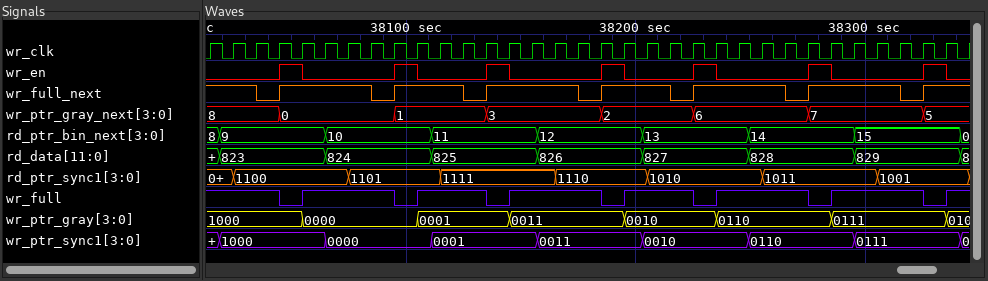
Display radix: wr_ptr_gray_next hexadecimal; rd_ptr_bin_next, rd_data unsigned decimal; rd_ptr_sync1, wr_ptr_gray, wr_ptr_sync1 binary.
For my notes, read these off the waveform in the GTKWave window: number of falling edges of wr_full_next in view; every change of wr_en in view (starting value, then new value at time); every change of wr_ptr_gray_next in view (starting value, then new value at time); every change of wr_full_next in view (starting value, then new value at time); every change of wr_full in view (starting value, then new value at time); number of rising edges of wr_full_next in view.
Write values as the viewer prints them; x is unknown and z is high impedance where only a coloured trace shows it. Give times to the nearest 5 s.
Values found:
7
0, 1 at 38045 s, 0 at 38055 s, 1 at 38095 s, 0 at 38105 s, 1 at 38135 s, 0 at 38145 s, 1 at 38185 s, 0 at 38195 s, 1 at 38225 s, 0 at 38235 s, 1 at 38275 s, 0 at 38285 s, 1 at 38325 s, 0 at 38335 s
8, 0 at 38045 s, 1 at 38095 s, 3 at 38135 s, 2 at 38185 s, 6 at 38225 s, 7 at 38275 s, 5 at 38325 s
1, 0 at 38035 s, 1 at 38045 s, 0 at 38085 s, 1 at 38095 s, 0 at 38125 s, 1 at 38135 s, 0 at 38175 s, 1 at 38185 s, 0 at 38215 s, 1 at 38225 s, 0 at 38265 s, 1 at 38275 s, 0 at 38315 s, 1 at 38325 s
1, 0 at 38045 s, 1 at 38055 s, 0 at 38095 s, 1 at 38105 s, 0 at 38135 s, 1 at 38145 s, 0 at 38185 s, 1 at 38195 s, 0 at 38225 s, 1 at 38235 s, 0 at 38275 s, 1 at 38285 s, 0 at 38325 s, 1 at 38335 s
7
